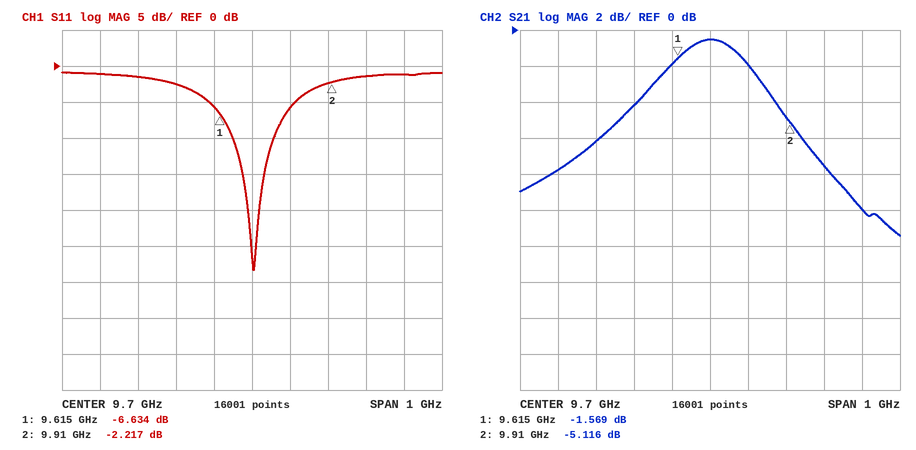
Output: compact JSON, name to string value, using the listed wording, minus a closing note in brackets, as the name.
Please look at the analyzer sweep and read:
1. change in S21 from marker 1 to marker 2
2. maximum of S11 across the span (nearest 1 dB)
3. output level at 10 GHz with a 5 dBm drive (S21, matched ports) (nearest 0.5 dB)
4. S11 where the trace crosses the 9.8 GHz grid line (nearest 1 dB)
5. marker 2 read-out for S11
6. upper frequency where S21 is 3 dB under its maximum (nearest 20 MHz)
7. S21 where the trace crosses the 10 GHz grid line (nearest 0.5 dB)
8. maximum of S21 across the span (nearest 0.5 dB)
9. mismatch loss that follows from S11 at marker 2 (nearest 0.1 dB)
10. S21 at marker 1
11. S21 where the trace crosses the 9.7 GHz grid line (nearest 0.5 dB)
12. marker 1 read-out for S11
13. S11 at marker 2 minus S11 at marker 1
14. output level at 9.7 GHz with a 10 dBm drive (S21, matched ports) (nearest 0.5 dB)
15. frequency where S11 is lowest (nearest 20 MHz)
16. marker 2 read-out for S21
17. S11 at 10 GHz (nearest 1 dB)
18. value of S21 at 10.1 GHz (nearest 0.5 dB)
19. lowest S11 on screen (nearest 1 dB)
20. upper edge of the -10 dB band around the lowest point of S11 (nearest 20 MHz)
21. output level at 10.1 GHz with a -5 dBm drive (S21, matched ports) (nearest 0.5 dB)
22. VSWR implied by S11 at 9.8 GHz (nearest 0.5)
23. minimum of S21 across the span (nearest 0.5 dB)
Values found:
{"change in S21 from marker 1 to marker 2": "-3.547 dB", "maximum of S11 across the span": "-1 dB", "output level at 10 GHz with a 5 dBm drive (S21, matched ports)": "-2.5 dBm", "S11 where the trace crosses the 9.8 GHz grid line": "-6 dB", "marker 2 read-out for S11": "-2.217 dB", "upper frequency where S21 is 3 dB under its maximum": "9.86 GHz", "S21 where the trace crosses the 10 GHz grid line": "-7.5 dB", "maximum of S21 across the span": "-0.5 dB", "mismatch loss that follows from S11 at marker 2": "4.0 dB", "S21 at marker 1": "-1.569 dB", "S21 where the trace crosses the 9.7 GHz grid line": "-0.5 dB", "marker 1 read-out for S11": "-6.634 dB", "S11 at marker 2 minus S11 at marker 1": "4.417 dB", "output level at 9.7 GHz with a 10 dBm drive (S21, matched ports)": "9.5 dBm", "frequency where S11 is lowest": "9.70 GHz", "marker 2 read-out for S21": "-5.116 dB", "S11 at 10 GHz": "-1 dB", "value of S21 at 10.1 GHz": "-10.0 dB", "lowest S11 on screen": "-28 dB", "upper edge of the -10 dB band around the lowest point of S11": "9.76 GHz", "output level at 10.1 GHz with a -5 dBm drive (S21, matched ports)": "-15.0 dBm", "VSWR implied by S11 at 9.8 GHz": "3.0", "minimum of S21 across the span": "-11.5 dB"}
